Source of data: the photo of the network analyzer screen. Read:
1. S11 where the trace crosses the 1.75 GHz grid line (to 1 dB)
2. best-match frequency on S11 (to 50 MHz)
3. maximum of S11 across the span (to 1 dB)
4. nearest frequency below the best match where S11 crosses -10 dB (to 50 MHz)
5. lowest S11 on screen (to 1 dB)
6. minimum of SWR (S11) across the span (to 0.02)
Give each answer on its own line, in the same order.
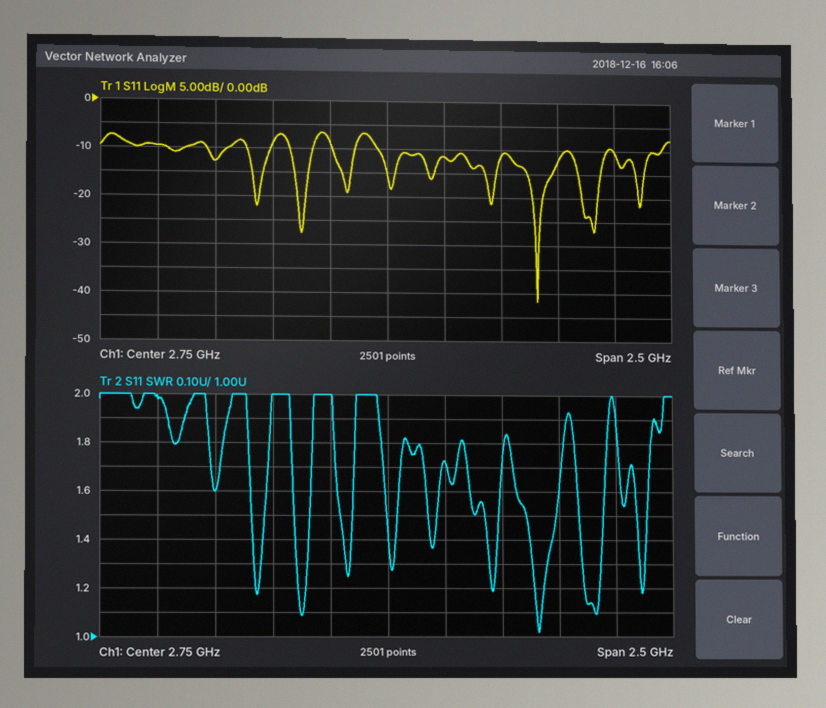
-10 dB
3.40 GHz
-7 dB
2.70 GHz
-42 dB
1.02
